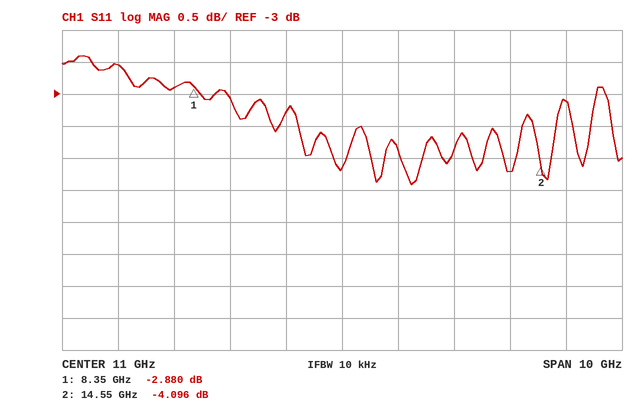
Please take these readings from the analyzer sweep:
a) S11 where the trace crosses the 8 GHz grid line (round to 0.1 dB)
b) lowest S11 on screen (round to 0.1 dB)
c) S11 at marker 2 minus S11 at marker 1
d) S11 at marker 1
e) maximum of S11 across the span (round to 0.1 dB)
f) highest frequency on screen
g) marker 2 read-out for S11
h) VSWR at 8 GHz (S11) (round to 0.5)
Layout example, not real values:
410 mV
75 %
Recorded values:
-2.9 dB
-4.4 dB
-1.216 dB
-2.880 dB
-2.4 dB
16 GHz
-4.096 dB
6.0
